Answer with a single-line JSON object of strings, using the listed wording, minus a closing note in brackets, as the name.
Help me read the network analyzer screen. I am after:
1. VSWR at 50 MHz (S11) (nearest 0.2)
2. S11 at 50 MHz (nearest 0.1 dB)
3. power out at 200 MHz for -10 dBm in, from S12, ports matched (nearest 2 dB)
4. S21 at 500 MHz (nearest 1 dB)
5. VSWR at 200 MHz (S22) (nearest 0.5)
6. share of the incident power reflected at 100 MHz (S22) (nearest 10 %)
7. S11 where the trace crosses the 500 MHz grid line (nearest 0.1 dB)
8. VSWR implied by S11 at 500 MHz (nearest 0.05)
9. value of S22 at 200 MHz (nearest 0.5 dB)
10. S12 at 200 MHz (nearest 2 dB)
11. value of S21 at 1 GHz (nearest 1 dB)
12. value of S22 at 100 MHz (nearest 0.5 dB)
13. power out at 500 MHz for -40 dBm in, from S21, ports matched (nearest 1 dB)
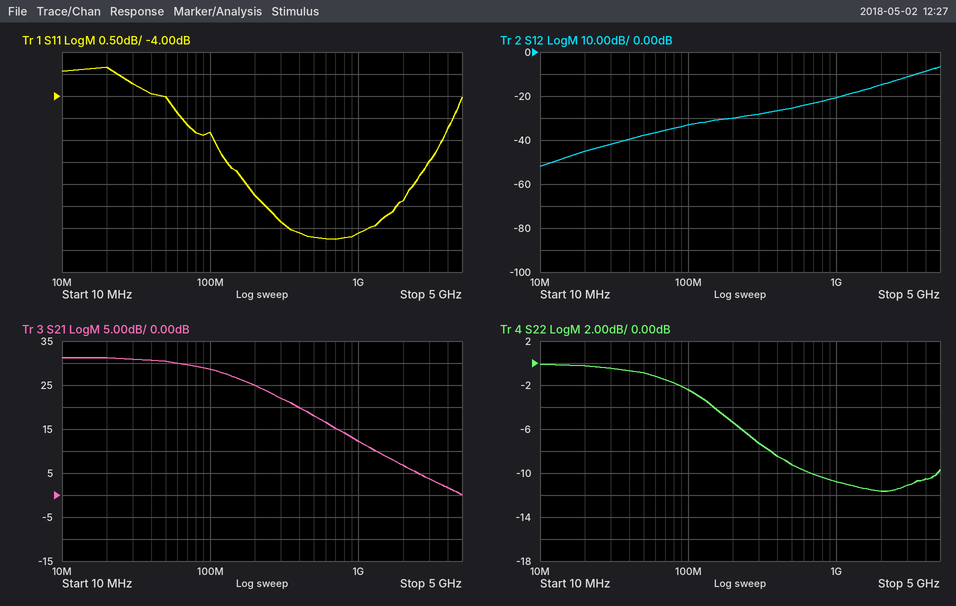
{"VSWR at 50 MHz (S11)": "4.4", "S11 at 50 MHz": "-4.0 dB", "power out at 200 MHz for -10 dBm in, from S12, ports matched": "-40 dBm", "S21 at 500 MHz": "18 dB", "VSWR at 200 MHz (S22)": "3.5", "share of the incident power reflected at 100 MHz (S22)": "60 %", "S11 where the trace crosses the 500 MHz grid line": "-7.2 dB", "VSWR implied by S11 at 500 MHz": "2.55", "value of S22 at 200 MHz": "-5.5 dB", "S12 at 200 MHz": "-30 dB", "value of S21 at 1 GHz": "12 dB", "value of S22 at 100 MHz": "-2.5 dB", "power out at 500 MHz for -40 dBm in, from S21, ports matched": "-22 dBm"}
